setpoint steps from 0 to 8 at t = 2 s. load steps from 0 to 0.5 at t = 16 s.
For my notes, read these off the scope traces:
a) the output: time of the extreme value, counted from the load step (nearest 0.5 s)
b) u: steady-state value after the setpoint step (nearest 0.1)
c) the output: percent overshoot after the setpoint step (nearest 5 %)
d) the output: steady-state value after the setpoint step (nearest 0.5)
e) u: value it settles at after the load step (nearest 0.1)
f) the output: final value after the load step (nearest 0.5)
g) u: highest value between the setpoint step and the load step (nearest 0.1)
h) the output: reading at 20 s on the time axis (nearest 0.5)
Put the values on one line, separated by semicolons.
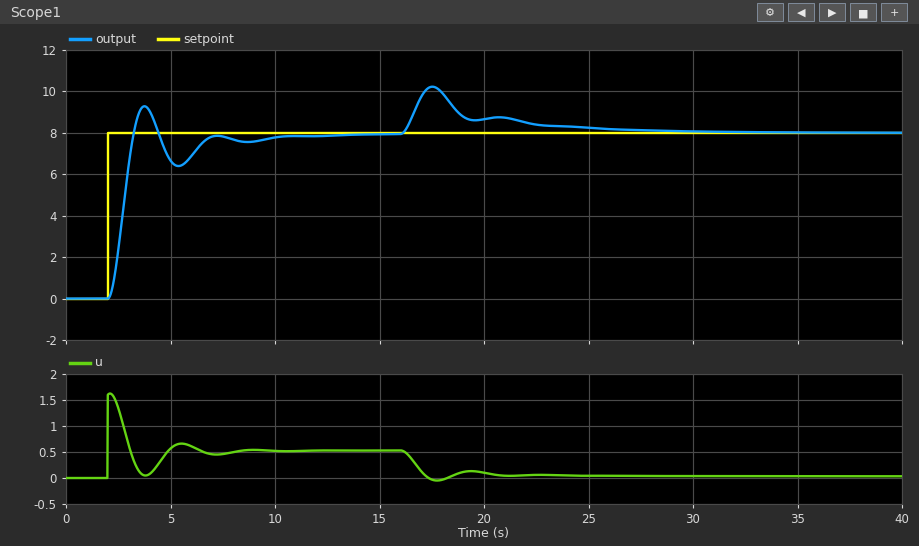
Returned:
1.5 s; 0.5; 15 %; 8.0; 0.0; 8.0; 1.6; 8.5
